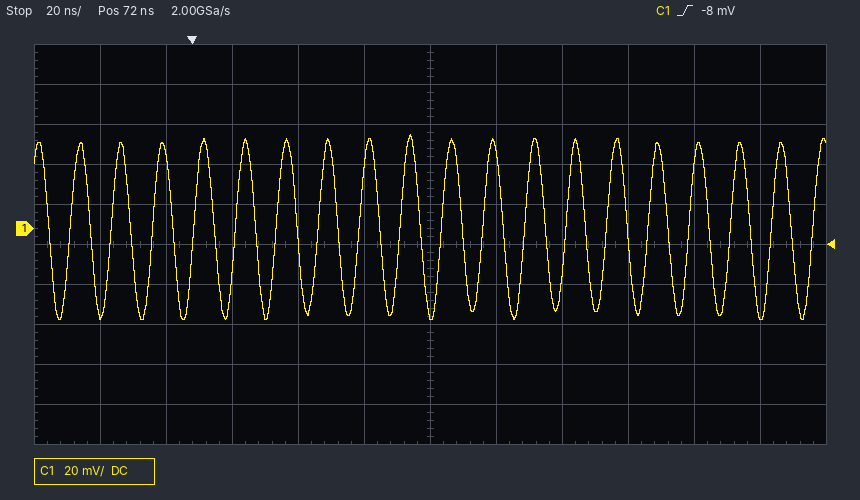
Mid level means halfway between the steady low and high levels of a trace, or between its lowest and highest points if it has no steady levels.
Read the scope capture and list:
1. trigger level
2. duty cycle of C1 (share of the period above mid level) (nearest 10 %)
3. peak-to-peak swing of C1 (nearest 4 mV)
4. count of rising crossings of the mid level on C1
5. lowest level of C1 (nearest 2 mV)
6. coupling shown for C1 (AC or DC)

-8 mV
50 %
92 mV
19
-46 mV
DC
